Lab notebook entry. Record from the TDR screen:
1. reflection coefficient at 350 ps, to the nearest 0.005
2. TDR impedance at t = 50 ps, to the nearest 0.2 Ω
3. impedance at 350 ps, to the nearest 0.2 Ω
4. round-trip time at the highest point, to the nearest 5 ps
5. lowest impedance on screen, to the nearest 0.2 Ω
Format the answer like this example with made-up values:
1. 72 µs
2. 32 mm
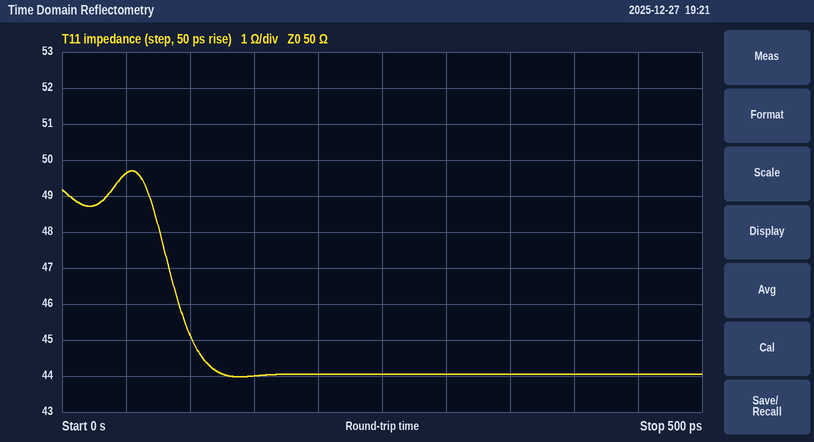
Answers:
1. -0.065
2. 49.6 Ω
3. 44.0 Ω
4. 55 ps
5. 44.0 Ω
